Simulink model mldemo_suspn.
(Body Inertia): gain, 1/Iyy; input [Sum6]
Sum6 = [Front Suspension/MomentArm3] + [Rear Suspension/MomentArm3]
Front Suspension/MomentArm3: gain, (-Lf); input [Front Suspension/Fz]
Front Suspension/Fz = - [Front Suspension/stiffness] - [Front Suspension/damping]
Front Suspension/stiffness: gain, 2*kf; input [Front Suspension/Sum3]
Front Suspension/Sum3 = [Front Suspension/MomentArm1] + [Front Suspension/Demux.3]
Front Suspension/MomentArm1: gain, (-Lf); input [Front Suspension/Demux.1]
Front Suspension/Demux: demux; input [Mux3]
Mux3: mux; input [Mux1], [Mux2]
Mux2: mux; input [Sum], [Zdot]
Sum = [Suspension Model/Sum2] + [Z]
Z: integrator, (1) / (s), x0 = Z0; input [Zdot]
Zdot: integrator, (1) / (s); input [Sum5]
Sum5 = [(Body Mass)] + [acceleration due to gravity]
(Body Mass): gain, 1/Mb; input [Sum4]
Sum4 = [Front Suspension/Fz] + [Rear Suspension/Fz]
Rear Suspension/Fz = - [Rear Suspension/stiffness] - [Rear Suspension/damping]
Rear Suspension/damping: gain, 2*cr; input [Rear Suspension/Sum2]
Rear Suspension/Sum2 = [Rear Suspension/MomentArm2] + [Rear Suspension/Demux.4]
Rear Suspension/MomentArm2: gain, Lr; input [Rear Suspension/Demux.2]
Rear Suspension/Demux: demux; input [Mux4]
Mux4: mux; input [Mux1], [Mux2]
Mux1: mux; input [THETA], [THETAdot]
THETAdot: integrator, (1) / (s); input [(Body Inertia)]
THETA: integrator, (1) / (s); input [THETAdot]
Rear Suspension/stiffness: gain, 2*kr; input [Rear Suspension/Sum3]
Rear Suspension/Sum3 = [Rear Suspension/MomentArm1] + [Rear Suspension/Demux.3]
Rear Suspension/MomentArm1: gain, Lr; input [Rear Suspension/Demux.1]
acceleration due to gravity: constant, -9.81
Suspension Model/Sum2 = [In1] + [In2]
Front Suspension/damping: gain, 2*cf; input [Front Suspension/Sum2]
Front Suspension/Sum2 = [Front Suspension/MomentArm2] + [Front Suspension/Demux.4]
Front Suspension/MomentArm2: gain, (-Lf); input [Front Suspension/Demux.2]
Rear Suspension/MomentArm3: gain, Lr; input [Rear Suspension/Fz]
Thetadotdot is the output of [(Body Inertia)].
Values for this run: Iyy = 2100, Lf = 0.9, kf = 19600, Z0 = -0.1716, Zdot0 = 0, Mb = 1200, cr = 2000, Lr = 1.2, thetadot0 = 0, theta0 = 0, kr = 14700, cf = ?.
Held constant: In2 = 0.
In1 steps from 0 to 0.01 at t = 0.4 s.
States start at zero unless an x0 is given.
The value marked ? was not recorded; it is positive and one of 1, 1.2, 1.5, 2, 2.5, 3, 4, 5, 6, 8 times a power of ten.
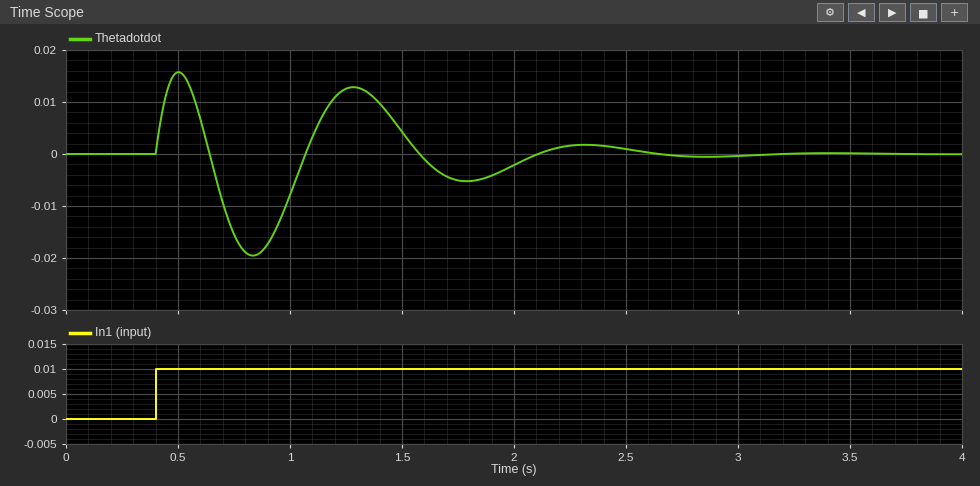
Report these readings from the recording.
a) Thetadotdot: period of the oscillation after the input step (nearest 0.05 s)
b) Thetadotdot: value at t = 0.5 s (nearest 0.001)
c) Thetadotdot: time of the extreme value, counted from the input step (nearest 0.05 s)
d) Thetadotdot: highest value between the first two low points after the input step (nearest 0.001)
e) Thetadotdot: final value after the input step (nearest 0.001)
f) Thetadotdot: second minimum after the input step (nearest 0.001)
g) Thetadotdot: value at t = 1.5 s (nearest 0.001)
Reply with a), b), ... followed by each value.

a) 0.95 s
b) 0.016
c) 0.45 s
d) 0.013
e) 0.000
f) -0.005
g) 0.004
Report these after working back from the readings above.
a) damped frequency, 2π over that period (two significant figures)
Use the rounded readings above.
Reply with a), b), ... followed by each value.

a) 6.6 rad/s
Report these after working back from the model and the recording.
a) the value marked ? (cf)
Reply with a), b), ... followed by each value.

a) 2000
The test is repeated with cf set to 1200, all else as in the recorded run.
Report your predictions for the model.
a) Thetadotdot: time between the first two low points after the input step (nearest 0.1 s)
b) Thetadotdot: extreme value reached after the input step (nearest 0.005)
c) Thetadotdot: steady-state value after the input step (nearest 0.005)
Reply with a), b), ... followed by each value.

a) 0.9 s
b) -0.055
c) 0.000
